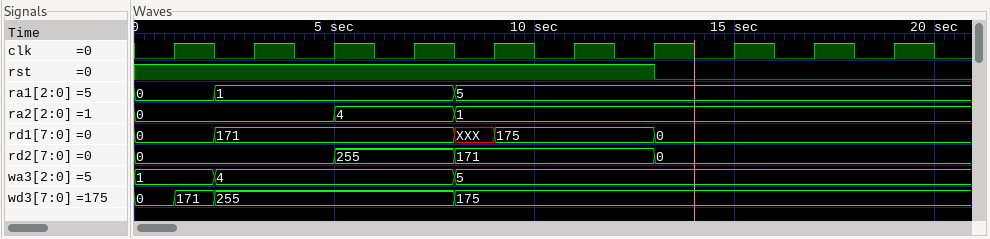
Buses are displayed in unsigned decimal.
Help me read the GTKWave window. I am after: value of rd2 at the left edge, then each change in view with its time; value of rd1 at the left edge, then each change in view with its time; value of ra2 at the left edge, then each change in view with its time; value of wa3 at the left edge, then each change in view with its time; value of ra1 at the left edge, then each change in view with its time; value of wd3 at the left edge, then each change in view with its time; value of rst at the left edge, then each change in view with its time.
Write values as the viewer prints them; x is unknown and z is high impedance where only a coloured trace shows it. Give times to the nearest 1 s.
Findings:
0, 255 at 5 s, 171 at 8 s, 0 at 13 s
0, 171 at 2 s, XXX at 8 s, 175 at 9 s, 0 at 13 s
0, 4 at 5 s, 1 at 8 s
1, 4 at 2 s, 5 at 8 s
0, 1 at 2 s, 5 at 8 s
0, 171 at 1 s, 255 at 2 s, 175 at 8 s
1, 0 at 13 s
